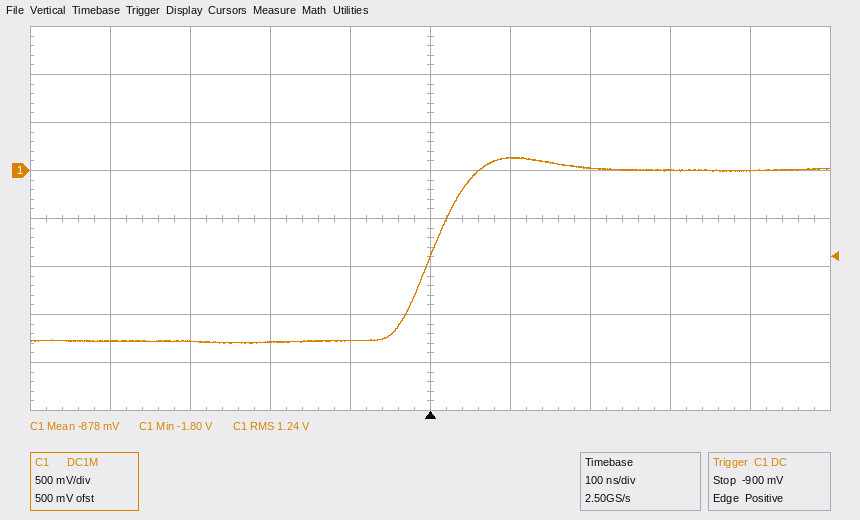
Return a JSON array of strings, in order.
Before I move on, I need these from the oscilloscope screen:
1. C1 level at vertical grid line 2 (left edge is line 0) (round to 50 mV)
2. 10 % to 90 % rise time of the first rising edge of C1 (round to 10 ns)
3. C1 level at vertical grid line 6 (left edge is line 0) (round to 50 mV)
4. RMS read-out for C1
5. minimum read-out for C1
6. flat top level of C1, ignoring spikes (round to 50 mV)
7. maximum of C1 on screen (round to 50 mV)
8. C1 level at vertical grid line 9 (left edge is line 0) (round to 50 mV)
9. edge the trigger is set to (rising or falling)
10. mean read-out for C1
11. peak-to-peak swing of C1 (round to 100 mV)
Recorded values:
["-1.80 V", "80 ns", "150 mV", "1.24 V", "-1.80 V", "0 mV", "150 mV", "0 mV", "rising", "-878 mV", "1.90 V"]
